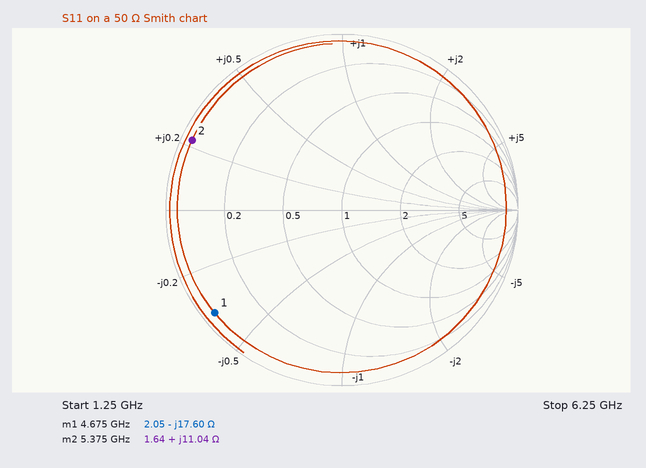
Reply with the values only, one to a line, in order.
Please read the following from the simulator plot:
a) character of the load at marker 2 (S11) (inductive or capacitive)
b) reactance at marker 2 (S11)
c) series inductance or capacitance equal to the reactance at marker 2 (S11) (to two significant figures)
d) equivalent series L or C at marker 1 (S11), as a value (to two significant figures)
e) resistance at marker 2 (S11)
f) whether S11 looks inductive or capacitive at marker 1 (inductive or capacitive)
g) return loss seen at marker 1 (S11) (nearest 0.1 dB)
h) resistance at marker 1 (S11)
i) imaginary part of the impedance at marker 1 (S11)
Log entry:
inductive
+11.04 Ω
330 pH
1.9 pF
1.64 Ω
capacitive
0.6 dB
2.05 Ω
-17.60 Ω
